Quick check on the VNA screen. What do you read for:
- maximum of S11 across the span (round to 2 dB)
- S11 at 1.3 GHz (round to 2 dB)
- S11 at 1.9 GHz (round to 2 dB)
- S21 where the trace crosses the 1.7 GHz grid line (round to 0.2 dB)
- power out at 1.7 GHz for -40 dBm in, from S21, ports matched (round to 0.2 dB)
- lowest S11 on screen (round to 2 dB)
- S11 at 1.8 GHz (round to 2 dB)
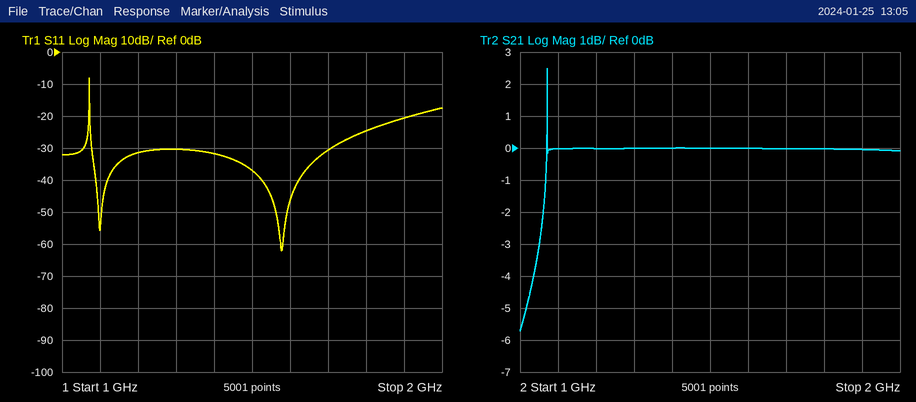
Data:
-8 dB
-30 dB
-20 dB
0.0 dB
-40.0 dBm
-62 dB
-24 dB
